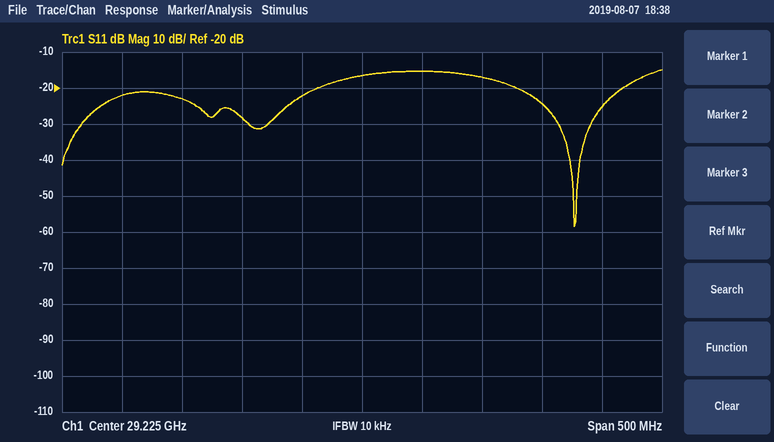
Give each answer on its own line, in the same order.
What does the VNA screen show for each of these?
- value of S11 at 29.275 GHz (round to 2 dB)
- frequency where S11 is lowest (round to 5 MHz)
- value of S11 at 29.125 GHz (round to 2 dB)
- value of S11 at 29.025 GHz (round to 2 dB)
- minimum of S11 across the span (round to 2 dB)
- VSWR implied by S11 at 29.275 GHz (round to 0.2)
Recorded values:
-16 dB
29.400 GHz
-28 dB
-22 dB
-58 dB
1.4
